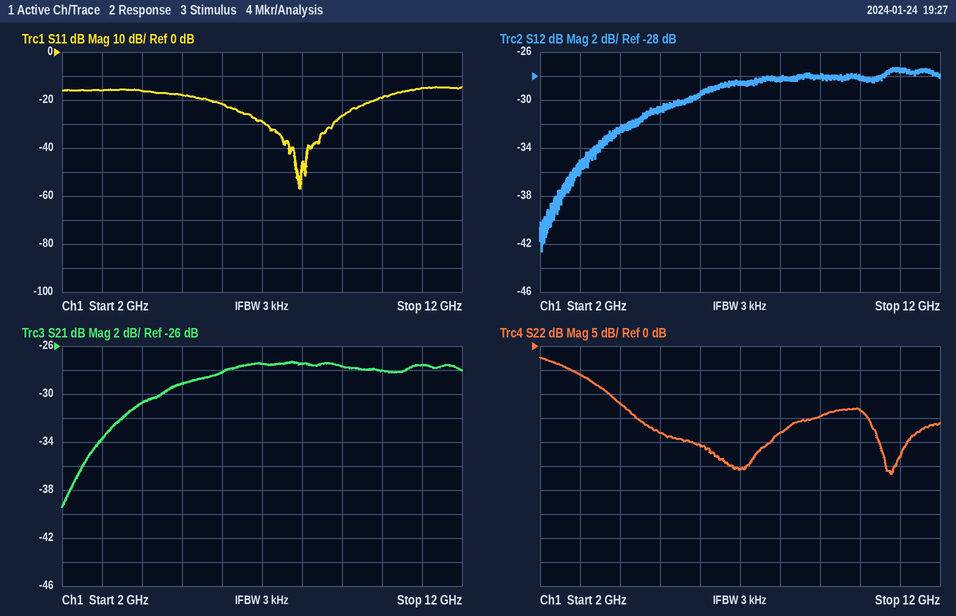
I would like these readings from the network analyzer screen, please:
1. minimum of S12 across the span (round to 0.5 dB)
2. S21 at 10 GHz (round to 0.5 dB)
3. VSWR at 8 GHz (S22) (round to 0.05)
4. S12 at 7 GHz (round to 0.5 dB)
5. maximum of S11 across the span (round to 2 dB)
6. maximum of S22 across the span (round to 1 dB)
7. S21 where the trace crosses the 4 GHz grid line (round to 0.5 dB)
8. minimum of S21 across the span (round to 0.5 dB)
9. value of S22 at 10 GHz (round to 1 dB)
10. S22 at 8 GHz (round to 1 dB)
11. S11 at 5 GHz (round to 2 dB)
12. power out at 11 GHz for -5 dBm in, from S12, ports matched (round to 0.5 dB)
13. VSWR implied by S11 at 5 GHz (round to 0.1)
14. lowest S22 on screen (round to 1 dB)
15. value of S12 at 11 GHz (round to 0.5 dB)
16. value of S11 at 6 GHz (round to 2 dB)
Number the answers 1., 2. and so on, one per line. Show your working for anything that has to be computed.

1. -42.5 dB
2. -28.0 dB
3. |Γ| = 10^(-18/20) = 0.1259; VSWR = (1 + 0.1259)/(1 − 0.1259) ≈ 1.29, so 1.30 to the nearest 0.05
4. -28.5 dB
5. -14 dB
6. -2 dB
7. -30.5 dB
8. -39.5 dB
9. -13 dB
10. -18 dB
11. -18 dB
12. -5 dBm + (-27.5 dB) = -32.5 dBm
13. |Γ| = 10^(-18/20) = 0.1259; VSWR = (1 + 0.1259)/(1 − 0.1259) ≈ 1.3
14. -27 dB
15. -27.5 dB
16. -22 dB
